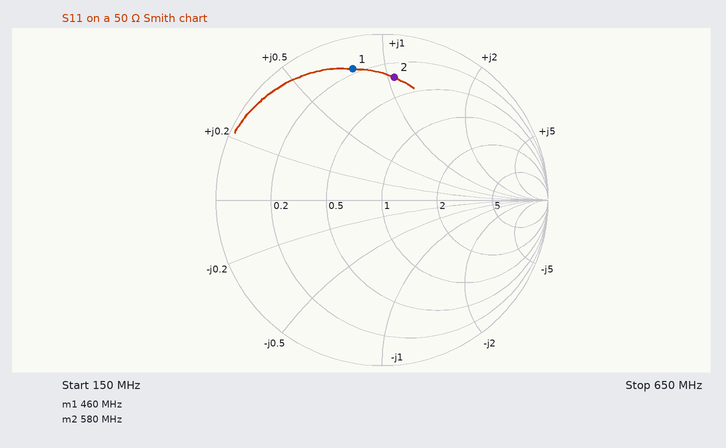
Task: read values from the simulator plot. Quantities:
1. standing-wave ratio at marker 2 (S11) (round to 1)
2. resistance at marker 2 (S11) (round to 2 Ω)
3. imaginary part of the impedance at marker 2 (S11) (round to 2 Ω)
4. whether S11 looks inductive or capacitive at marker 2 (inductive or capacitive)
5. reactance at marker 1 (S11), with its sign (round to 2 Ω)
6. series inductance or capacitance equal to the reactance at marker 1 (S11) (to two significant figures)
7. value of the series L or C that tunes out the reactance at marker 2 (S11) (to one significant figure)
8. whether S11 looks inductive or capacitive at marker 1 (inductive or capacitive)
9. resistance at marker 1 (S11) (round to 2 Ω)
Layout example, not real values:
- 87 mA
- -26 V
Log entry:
- 7
- 16 Ω
- +52 Ω
- inductive
- +40 Ω
- 14 nH
- 5 pF
- inductive
- 8 Ω
